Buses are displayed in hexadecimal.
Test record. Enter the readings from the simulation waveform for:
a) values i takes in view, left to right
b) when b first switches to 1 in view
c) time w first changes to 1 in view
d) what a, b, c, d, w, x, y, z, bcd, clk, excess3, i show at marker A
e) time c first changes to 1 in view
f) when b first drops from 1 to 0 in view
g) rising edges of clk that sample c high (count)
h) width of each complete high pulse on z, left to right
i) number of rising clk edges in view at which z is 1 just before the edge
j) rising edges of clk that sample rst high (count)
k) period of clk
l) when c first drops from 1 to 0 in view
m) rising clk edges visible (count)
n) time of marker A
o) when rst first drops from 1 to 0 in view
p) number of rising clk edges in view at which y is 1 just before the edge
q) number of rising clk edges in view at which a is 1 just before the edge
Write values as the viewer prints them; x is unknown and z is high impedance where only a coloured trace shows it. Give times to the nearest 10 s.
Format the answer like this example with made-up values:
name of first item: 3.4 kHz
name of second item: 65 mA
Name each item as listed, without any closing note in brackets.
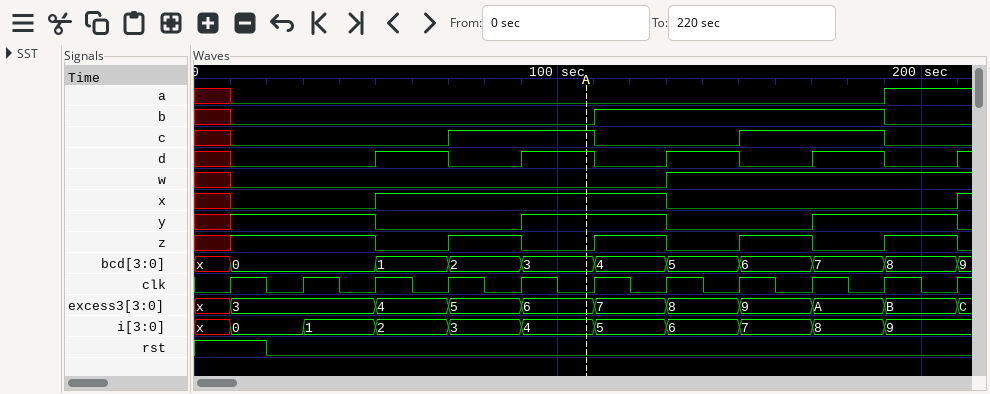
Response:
values i takes in view, left to right: x, 0, 1, 2, 3, 4, 5, 6, 7, 8, 9
when b first switches to 1 in view: 110 s
time w first changes to 1 in view: 130 s
what a, b, c, d, w, x, y, z, bcd, clk, excess3, i show at marker A: a=0, b=0, c=1, d=1, w=0, x=1, y=1, z=0, bcd=3, clk=0, excess3=6, i=4
time c first changes to 1 in view: 70 s
when b first drops from 1 to 0 in view: 190 s
rising edges of clk that sample c high: 4
width of each complete high pulse on z, left to right: 20 s, 20 s, 20 s, 20 s
number of rising clk edges in view at which z is 1 just before the edge: 6
rising edges of clk that sample rst high: 1
period of clk: 20 s
when c first drops from 1 to 0 in view: 110 s
rising clk edges visible: 11
time of marker A: 110 s
when rst first drops from 1 to 0 in view: 20 s
number of rising clk edges in view at which y is 1 just before the edge: 6
number of rising clk edges in view at which a is 1 just before the edge: 1
